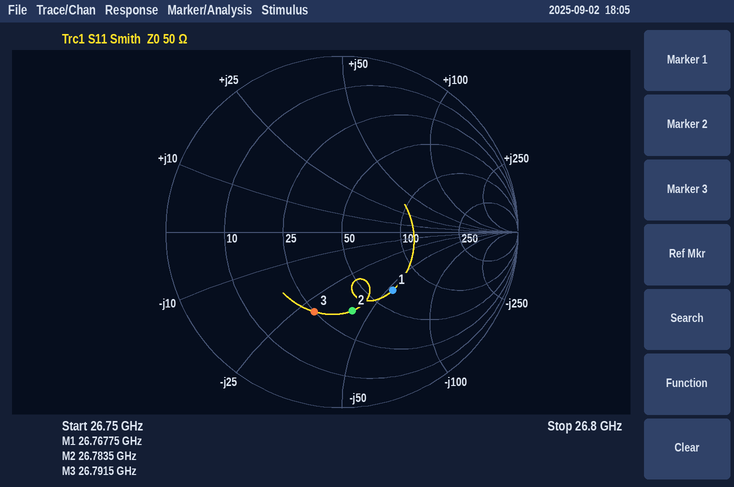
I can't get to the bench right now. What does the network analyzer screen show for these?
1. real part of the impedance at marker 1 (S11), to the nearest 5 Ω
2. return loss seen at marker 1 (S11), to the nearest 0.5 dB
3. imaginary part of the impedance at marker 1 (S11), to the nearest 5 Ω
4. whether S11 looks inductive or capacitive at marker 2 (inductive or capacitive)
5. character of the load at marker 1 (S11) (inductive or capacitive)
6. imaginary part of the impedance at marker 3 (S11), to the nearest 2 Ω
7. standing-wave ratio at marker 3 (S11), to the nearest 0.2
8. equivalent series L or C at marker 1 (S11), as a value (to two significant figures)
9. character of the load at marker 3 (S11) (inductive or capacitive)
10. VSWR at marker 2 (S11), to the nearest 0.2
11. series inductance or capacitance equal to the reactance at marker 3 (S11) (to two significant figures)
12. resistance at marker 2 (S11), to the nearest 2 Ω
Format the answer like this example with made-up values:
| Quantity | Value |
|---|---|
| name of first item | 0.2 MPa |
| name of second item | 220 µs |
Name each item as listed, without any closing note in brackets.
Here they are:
| Quantity | Value |
|---|---|
| real part of the impedance at marker 1 (S11), to the nearest 5 Ω | 65 Ω |
| return loss seen at marker 1 (S11), to the nearest 0.5 dB | 7.0 dB |
| imaginary part of the impedance at marker 1 (S11), to the nearest 5 Ω | -55 Ω |
| whether S11 looks inductive or capacitive at marker 2 | capacitive |
| character of the load at marker 1 (S11) | capacitive |
| imaginary part of the impedance at marker 3 (S11), to the nearest 2 Ω | -30 Ω |
| standing-wave ratio at marker 3 (S11), to the nearest 0.2 | 2.8 |
| equivalent series L or C at marker 1 (S11), as a value | 110 fF |
| character of the load at marker 3 (S11) | capacitive |
| VSWR at marker 2 (S11), to the nearest 0.2 | 2.6 |
| series inductance or capacitance equal to the reactance at marker 3 (S11) | 200 fF |
| resistance at marker 2 (S11), to the nearest 2 Ω | 36 Ω |
